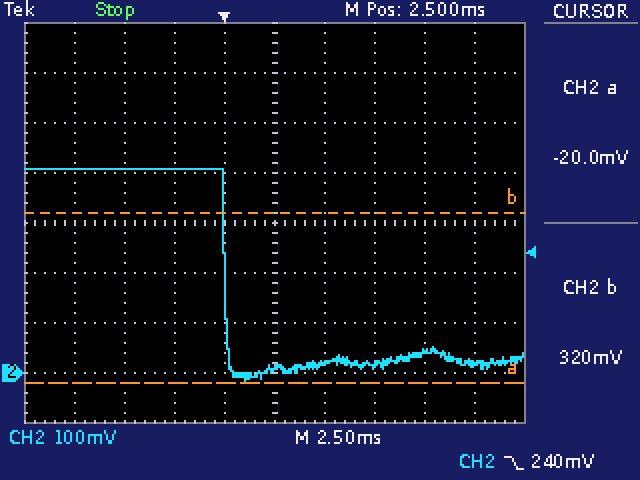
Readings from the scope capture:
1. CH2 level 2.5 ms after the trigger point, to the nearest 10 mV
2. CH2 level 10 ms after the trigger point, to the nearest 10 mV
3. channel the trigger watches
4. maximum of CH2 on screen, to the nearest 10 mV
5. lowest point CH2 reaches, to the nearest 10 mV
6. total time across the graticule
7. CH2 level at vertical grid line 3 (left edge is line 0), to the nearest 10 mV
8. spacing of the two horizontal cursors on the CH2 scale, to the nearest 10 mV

10 mV
40 mV
CH2
410 mV
-20 mV
25 ms
410 mV
340 mV
